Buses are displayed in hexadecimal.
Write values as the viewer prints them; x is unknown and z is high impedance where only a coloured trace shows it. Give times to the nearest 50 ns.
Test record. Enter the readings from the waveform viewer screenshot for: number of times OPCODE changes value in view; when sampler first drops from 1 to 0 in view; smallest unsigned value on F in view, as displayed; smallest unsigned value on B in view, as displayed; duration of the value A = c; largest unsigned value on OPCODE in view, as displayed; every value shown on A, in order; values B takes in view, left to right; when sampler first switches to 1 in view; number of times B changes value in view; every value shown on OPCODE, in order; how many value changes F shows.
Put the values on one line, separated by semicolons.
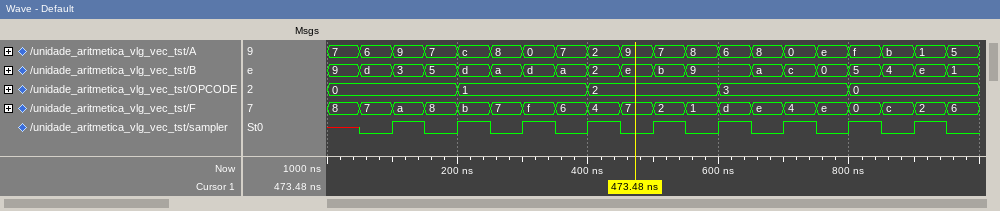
4; 150 ns; 0; 0; 50 ns; 3; 7, 6, 9, 7, c, 8, 0, 7, 2, 9, 7, 8, 6, 8, 0, e, f, b, 1, 5; 9, d, 3, 5, d, a, d, a, 2, e, b, 9, a, c, 0, 5, 4, e, 1; 100 ns; 18; 0, 1, 2, 3, 0; 19
